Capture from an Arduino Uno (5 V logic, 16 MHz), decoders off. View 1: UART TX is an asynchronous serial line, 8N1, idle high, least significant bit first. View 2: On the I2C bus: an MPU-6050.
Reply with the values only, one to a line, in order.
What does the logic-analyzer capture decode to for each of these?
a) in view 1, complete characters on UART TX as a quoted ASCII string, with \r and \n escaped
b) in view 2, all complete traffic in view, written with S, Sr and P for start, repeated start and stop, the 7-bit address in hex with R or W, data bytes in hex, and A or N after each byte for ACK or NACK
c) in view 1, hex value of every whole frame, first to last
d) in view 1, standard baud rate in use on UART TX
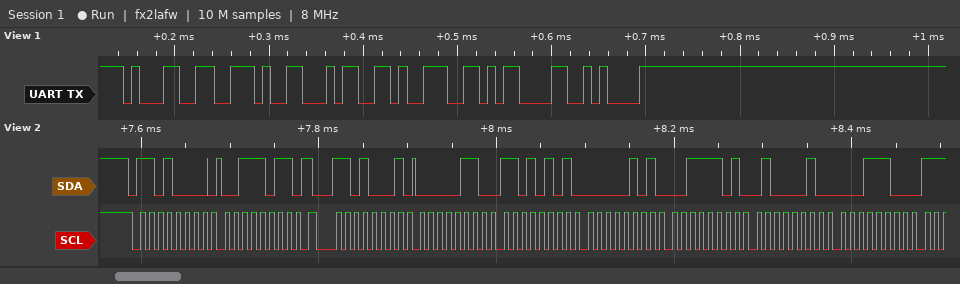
"1.49\r\n"
S 68W A 3B A Sr 68R A 06 A D5 A 05 A 3D A 42 A 1C A
31 2E 34 39 0D 0A
115200 baud
